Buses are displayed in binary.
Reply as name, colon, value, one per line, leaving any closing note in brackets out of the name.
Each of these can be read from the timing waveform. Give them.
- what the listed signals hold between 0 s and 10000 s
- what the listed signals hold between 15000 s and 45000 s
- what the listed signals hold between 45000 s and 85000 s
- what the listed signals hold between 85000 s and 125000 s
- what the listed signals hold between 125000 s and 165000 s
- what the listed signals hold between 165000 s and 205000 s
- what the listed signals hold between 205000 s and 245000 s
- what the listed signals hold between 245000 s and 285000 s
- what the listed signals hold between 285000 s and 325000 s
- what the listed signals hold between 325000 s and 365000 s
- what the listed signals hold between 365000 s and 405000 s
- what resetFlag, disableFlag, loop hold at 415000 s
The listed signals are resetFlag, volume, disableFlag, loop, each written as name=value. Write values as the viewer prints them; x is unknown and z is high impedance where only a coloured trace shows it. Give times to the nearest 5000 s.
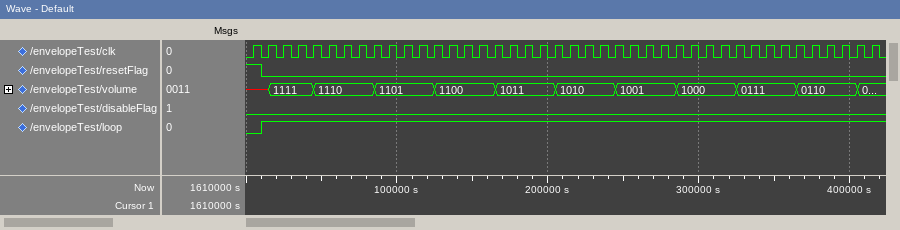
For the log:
what the listed signals hold between 0 s and 10000 s: resetFlag=1, volume=x, disableFlag=0, loop=0
what the listed signals hold between 15000 s and 45000 s: resetFlag=0, volume=1111, disableFlag=0, loop=1
what the listed signals hold between 45000 s and 85000 s: resetFlag=0, volume=1110, disableFlag=0, loop=1
what the listed signals hold between 85000 s and 125000 s: resetFlag=0, volume=1101, disableFlag=0, loop=1
what the listed signals hold between 125000 s and 165000 s: resetFlag=0, volume=1100, disableFlag=0, loop=1
what the listed signals hold between 165000 s and 205000 s: resetFlag=0, volume=1011, disableFlag=0, loop=1
what the listed signals hold between 205000 s and 245000 s: resetFlag=0, volume=1010, disableFlag=0, loop=1
what the listed signals hold between 245000 s and 285000 s: resetFlag=0, volume=1001, disableFlag=0, loop=1
what the listed signals hold between 285000 s and 325000 s: resetFlag=0, volume=1000, disableFlag=0, loop=1
what the listed signals hold between 325000 s and 365000 s: resetFlag=0, volume=0111, disableFlag=0, loop=1
what the listed signals hold between 365000 s and 405000 s: resetFlag=0, volume=0110, disableFlag=0, loop=1
what resetFlag, disableFlag, loop hold at 415000 s: resetFlag=0, disableFlag=0, loop=1
